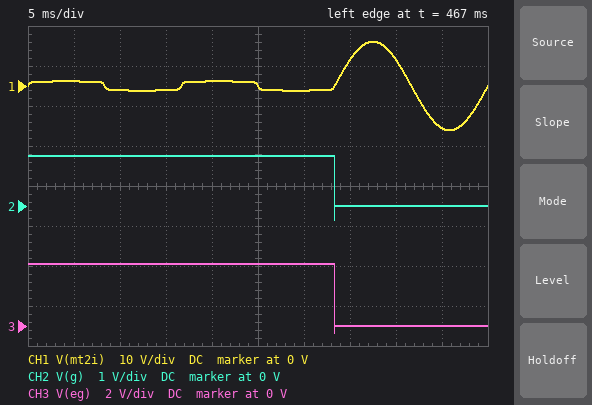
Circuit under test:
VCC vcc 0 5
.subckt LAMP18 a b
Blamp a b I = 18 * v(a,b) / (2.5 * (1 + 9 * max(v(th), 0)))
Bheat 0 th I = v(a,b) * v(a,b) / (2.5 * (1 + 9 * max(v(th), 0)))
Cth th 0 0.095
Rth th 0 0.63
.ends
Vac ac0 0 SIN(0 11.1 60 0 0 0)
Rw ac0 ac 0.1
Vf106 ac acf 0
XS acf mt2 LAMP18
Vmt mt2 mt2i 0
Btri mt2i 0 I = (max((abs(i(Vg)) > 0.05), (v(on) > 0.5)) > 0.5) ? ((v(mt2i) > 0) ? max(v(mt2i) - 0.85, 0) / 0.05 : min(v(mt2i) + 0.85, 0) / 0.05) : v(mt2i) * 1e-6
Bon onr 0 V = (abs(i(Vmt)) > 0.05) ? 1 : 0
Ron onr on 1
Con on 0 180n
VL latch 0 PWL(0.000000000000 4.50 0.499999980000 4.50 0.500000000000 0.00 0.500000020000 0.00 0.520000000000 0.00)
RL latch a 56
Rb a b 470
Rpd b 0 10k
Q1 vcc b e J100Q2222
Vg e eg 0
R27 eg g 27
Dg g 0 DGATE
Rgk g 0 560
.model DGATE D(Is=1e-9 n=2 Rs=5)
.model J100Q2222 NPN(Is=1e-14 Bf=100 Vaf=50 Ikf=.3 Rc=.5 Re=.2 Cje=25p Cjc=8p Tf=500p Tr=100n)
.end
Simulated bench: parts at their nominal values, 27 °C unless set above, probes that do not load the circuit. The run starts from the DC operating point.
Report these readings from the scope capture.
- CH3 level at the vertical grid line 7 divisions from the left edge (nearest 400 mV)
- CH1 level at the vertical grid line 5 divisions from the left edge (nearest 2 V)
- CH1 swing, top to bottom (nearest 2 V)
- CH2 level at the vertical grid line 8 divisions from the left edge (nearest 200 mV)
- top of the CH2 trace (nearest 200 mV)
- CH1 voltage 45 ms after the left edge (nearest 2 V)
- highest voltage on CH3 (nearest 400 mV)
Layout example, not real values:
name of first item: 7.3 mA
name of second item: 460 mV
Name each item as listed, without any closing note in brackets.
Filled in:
CH3 level at the vertical grid line 7 divisions from the left edge: 0 V
CH1 level at the vertical grid line 5 divisions from the left edge: 0 V
CH1 swing, top to bottom: 22 V
CH2 level at the vertical grid line 8 divisions from the left edge: 0 V
top of the CH2 trace: 1.2 V
CH1 voltage 45 ms after the left edge: -10 V
highest voltage on CH3: 3.2 V
